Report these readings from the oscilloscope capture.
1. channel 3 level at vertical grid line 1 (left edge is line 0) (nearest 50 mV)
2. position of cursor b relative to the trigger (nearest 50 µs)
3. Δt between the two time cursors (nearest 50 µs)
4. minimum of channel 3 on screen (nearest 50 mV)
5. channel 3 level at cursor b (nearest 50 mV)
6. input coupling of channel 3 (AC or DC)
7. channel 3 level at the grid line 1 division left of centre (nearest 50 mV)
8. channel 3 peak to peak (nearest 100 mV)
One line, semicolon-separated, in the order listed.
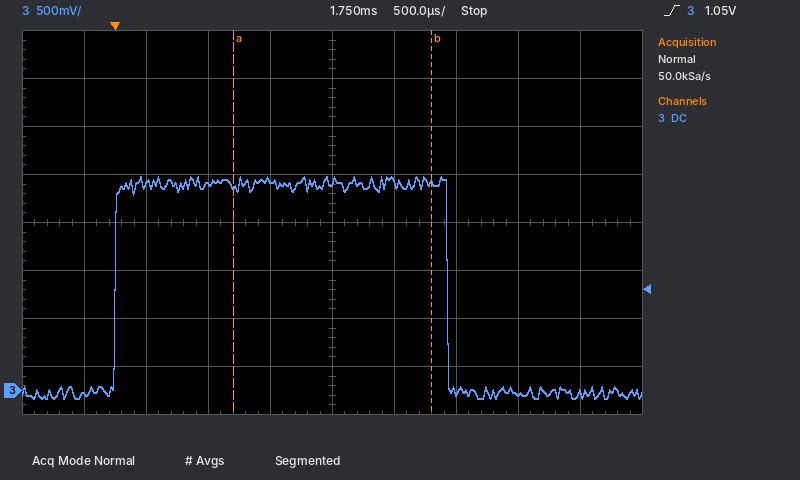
-50 mV; +2.55 ms; 1.60 ms; -100 mV; 2.15 V; DC; 2.20 V; 2.30 V
